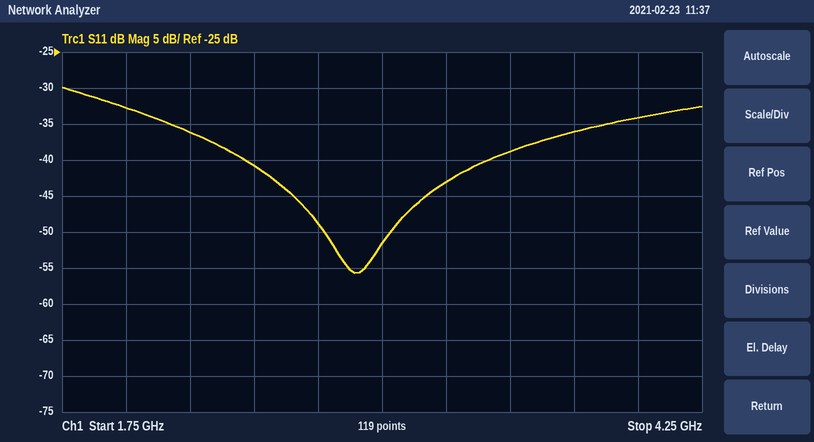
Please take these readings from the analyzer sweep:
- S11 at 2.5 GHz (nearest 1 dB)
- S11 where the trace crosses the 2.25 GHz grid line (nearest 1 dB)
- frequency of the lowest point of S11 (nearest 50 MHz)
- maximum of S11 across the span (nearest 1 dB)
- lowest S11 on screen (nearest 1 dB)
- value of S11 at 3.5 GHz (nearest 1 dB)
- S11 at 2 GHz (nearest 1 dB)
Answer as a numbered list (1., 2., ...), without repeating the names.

1. -41 dB
2. -36 dB
3. 2.90 GHz
4. -30 dB
5. -56 dB
6. -39 dB
7. -33 dB
